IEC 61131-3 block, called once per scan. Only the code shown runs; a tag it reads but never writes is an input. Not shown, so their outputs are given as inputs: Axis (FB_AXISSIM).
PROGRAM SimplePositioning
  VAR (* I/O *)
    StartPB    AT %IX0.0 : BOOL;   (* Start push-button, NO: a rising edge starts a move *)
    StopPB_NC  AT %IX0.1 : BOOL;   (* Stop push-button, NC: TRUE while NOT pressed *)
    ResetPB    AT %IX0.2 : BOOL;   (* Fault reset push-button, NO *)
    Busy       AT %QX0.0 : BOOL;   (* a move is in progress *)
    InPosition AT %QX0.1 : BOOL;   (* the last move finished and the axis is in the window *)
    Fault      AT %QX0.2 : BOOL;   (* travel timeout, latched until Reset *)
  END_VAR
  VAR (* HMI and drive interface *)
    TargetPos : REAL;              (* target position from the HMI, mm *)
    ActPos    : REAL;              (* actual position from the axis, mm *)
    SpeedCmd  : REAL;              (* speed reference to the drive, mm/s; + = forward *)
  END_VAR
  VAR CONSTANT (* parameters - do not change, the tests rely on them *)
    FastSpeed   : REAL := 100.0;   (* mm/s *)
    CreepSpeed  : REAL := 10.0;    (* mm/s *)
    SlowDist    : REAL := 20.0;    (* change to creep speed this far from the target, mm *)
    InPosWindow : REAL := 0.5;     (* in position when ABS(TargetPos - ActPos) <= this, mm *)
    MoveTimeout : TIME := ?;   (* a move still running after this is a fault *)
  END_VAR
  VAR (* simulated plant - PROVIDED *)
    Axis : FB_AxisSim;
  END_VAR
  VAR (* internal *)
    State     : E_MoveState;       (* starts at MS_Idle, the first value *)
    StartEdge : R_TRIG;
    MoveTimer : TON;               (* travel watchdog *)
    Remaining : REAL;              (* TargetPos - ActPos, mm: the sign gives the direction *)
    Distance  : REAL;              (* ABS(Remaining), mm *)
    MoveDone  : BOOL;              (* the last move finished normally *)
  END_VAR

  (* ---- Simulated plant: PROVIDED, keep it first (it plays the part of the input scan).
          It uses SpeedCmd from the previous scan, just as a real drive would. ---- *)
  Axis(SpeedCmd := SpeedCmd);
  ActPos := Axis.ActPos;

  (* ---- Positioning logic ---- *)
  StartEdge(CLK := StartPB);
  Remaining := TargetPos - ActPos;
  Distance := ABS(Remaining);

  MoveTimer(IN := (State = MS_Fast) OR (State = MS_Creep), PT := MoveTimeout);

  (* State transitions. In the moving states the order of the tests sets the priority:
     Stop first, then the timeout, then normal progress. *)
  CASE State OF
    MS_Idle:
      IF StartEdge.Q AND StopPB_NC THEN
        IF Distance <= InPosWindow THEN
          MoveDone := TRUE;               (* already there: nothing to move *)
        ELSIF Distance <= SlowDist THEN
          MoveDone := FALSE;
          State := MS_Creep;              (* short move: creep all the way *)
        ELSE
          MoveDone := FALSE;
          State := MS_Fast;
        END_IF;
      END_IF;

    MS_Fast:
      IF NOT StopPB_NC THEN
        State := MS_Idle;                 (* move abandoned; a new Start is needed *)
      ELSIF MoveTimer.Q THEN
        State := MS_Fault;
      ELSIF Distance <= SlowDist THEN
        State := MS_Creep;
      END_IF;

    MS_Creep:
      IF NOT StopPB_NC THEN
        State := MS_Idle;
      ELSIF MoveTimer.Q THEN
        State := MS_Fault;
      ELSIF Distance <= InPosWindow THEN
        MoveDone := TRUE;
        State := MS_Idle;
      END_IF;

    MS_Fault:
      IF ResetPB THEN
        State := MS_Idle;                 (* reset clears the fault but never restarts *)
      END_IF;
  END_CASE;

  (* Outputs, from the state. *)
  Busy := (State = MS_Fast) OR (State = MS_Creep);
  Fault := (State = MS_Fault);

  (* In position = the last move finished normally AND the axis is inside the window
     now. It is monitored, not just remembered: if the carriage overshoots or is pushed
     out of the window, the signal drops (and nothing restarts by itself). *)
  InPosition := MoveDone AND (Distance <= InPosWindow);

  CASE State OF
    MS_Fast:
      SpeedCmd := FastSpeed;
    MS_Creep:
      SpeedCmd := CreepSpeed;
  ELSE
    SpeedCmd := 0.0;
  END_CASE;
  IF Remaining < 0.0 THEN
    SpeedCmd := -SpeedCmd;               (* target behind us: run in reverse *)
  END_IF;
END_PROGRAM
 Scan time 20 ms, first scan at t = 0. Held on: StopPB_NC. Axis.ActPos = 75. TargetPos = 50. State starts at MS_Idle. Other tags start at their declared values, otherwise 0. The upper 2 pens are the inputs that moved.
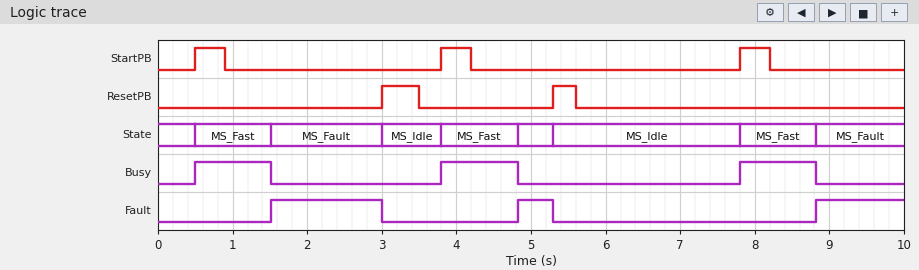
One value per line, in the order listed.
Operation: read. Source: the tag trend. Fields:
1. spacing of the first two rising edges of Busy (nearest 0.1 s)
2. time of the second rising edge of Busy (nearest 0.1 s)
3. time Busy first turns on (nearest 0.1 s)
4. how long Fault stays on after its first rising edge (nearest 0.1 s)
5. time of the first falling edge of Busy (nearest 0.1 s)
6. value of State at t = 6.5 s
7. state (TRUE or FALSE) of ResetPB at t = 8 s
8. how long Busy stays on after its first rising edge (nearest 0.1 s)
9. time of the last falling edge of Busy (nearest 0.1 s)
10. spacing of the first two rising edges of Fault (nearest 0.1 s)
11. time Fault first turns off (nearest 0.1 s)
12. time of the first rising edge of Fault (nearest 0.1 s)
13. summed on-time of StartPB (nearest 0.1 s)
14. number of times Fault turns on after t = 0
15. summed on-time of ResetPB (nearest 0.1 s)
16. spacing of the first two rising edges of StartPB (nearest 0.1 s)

3.3 s
3.8 s
0.5 s
1.5 s
1.5 s
MS_Idle
FALSE
1.0 s
8.8 s
3.3 s
3.0 s
1.5 s
1.2 s
3
0.8 s
3.3 s
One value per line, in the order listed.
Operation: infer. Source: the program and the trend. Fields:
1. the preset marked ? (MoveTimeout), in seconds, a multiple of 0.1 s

1.0 s
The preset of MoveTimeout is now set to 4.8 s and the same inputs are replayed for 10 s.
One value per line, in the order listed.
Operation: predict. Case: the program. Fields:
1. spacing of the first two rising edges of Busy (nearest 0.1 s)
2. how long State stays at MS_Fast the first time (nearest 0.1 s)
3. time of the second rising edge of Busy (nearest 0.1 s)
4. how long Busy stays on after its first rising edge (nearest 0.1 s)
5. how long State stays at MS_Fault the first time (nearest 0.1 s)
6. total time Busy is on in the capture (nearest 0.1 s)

7.3 s
4.8 s
7.8 s
4.8 s
0.0 s
7.0 s
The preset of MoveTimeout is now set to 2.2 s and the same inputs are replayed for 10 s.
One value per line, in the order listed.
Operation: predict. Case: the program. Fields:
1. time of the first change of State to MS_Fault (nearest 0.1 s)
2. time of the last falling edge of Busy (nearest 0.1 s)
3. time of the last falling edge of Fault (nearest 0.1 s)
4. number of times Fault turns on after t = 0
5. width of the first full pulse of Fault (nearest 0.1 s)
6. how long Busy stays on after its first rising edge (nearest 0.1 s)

2.7 s
6.0 s
3.0 s
2
0.3 s
2.2 s
